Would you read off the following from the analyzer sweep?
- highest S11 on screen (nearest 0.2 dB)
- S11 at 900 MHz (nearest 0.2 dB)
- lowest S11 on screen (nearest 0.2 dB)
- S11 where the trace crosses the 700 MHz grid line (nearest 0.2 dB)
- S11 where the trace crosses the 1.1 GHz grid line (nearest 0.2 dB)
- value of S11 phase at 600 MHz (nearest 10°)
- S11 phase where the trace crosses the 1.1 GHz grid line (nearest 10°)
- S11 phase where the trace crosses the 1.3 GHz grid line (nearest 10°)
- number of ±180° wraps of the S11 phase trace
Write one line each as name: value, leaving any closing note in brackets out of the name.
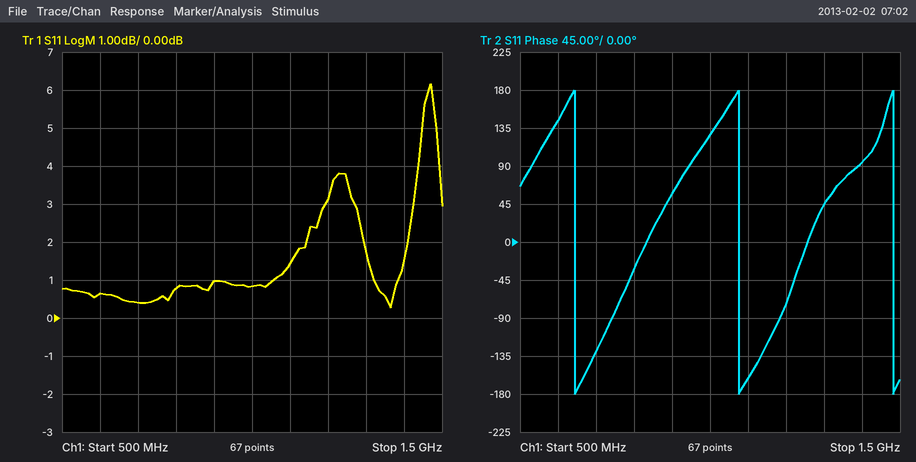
highest S11 on screen: 6.2 dB
S11 at 900 MHz: 1.0 dB
lowest S11 on screen: 0.2 dB
S11 where the trace crosses the 700 MHz grid line: 0.4 dB
S11 where the trace crosses the 1.1 GHz grid line: 1.4 dB
value of S11 phase at 600 MHz: 140°
S11 phase where the trace crosses the 1.1 GHz grid line: -160°
S11 phase where the trace crosses the 1.3 GHz grid line: 40°
number of ±180° wraps of the S11 phase trace: 3
